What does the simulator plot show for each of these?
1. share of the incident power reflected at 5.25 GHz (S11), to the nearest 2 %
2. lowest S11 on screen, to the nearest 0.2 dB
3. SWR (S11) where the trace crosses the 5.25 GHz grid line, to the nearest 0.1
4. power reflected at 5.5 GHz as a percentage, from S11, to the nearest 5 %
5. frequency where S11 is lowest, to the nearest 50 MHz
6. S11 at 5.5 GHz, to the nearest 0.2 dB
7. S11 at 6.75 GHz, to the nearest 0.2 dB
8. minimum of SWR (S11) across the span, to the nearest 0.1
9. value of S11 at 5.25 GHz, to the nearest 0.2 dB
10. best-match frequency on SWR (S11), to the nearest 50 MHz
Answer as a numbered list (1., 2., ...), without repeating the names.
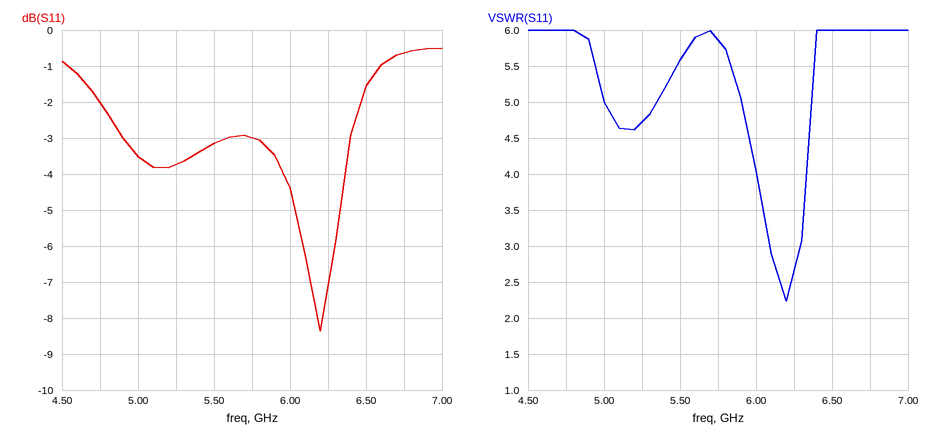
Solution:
1. 42 %
2. -8.4 dB
3. 4.7
4. 50 %
5. 6.20 GHz
6. -3.2 dB
7. -0.6 dB
8. 2.2
9. -3.8 dB
10. 6.20 GHz
